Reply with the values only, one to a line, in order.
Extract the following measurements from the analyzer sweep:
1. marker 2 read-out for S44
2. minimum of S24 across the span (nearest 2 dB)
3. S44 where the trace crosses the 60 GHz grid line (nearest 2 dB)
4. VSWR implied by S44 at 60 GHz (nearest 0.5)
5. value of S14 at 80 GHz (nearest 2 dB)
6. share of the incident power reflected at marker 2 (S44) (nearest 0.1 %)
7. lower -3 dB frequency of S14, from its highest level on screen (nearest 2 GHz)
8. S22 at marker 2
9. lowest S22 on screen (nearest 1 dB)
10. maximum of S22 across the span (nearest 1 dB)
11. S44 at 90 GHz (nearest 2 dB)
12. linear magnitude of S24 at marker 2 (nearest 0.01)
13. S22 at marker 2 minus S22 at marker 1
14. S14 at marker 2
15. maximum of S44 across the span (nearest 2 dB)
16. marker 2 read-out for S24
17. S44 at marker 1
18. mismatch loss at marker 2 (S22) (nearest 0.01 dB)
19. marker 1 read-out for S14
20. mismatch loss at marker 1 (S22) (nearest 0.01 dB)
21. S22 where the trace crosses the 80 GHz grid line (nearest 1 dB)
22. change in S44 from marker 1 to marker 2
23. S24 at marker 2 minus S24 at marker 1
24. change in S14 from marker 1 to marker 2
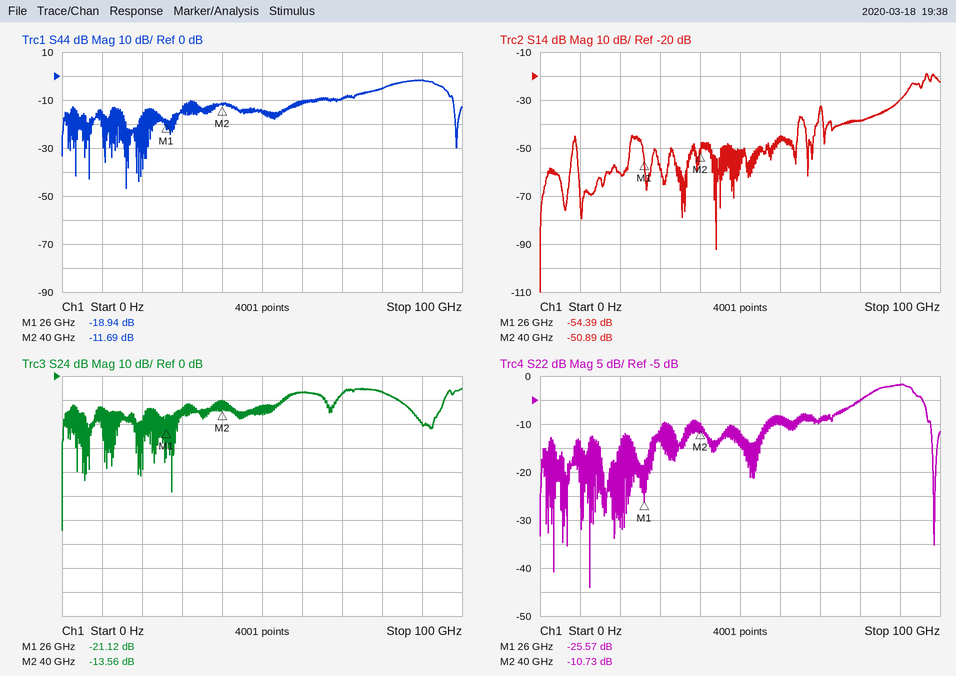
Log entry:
-11.69 dB
-64 dB
-10 dB
2.0
-38 dB
6.8 %
96 GHz
-10.73 dB
-44 dB
-2 dB
-2 dB
0.21
14.84 dB
-50.89 dB
-2 dB
-13.56 dB
-18.94 dB
0.38 dB
-54.39 dB
0.01 dB
-5 dB
7.25 dB
7.56 dB
3.50 dB
